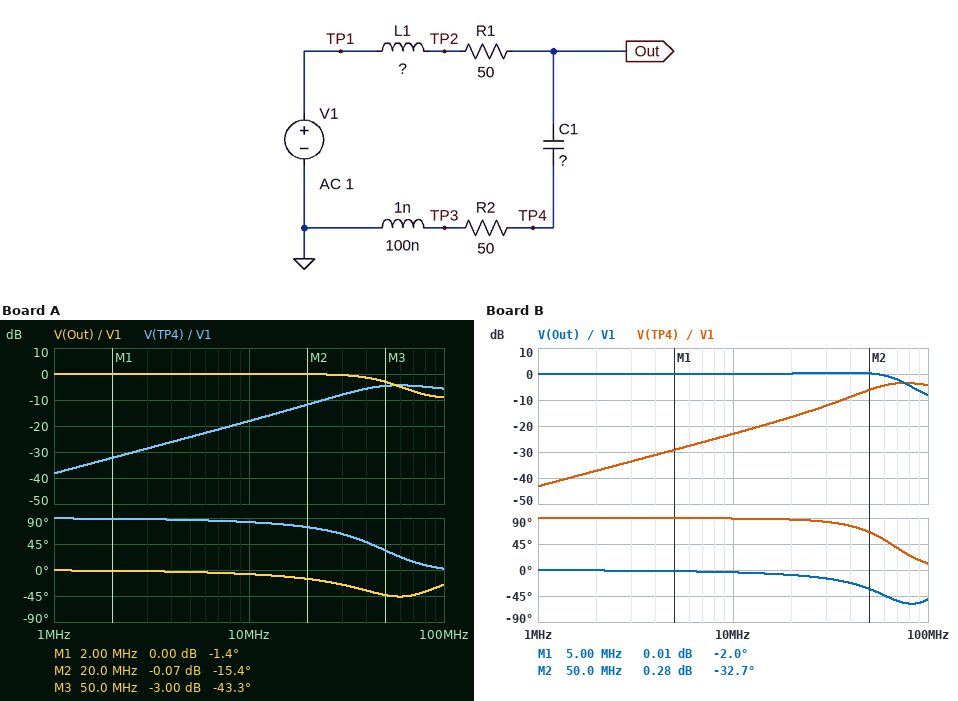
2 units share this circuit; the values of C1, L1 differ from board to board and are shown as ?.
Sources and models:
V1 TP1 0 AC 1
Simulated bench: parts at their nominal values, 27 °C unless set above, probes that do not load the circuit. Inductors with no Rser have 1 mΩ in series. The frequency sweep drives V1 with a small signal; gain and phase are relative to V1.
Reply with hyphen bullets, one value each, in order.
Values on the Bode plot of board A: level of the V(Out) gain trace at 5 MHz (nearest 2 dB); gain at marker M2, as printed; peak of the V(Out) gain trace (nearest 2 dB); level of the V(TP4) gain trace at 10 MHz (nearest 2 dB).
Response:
- 0 dB
- -0.07 dB
- 0 dB
- -18 dB
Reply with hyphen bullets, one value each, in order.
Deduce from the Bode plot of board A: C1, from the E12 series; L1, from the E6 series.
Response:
- 39 pF
- 150 nH
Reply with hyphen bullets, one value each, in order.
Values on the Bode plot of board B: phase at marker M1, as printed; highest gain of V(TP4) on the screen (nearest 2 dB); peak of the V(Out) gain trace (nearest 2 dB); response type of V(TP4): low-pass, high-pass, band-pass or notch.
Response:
- -2.0 deg
- -4 dB
- 0 dB
- high-pass
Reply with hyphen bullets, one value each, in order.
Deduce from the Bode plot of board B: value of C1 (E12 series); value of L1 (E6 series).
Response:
- 22 pF
- 150 nH
